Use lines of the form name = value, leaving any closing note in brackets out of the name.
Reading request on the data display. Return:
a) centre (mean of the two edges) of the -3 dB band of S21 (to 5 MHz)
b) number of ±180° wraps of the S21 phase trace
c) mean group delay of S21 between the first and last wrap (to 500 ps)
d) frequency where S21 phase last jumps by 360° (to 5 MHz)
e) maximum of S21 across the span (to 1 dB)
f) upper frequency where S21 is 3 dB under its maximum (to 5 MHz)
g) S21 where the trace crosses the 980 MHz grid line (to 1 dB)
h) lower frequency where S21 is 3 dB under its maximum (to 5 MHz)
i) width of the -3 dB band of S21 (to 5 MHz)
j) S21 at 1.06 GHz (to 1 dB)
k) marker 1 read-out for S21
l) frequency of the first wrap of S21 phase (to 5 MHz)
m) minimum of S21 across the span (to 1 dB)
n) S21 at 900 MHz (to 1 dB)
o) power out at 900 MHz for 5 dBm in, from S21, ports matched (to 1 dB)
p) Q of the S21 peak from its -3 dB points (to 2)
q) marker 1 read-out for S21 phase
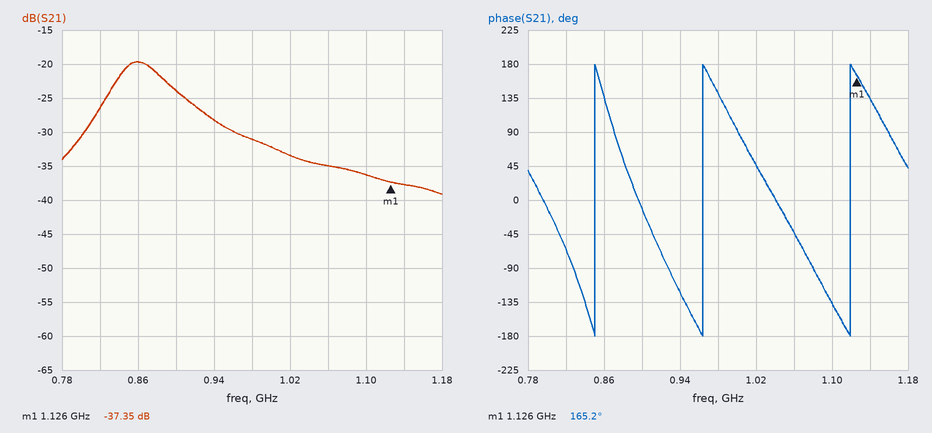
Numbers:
centre (mean of the two edges) of the -3 dB band of S21 = 865 MHz
number of ±180° wraps of the S21 phase trace = 3
mean group delay of S21 between the first and last wrap = 7.5 ns
frequency where S21 phase last jumps by 360° = 1.120 GHz
maximum of S21 across the span = -20 dB
upper frequency where S21 is 3 dB under its maximum = 890 MHz
S21 where the trace crosses the 980 MHz grid line = -31 dB
lower frequency where S21 is 3 dB under its maximum = 835 MHz
width of the -3 dB band of S21 = 55 MHz
S21 at 1.06 GHz = -35 dB
marker 1 read-out for S21 = -37.35 dB
frequency of the first wrap of S21 phase = 850 MHz
minimum of S21 across the span = -39 dB
S21 at 900 MHz = -24 dB
power out at 900 MHz for 5 dBm in, from S21, ports matched = -19 dBm
Q of the S21 peak from its -3 dB points = 16
marker 1 read-out for S21 phase = 165.2°
